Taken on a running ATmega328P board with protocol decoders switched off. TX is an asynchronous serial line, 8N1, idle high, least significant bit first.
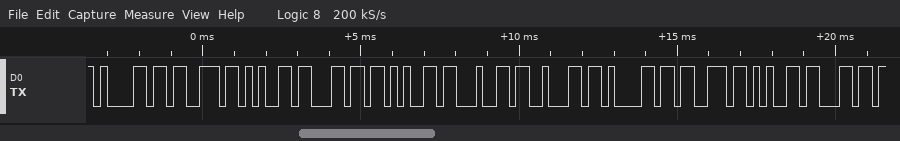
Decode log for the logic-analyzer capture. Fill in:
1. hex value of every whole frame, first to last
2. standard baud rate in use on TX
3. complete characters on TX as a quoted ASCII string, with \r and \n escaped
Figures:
0x61 0x73 0x65 0x6C 0x65 0x64 0x62 0x61 0x73 0x65 0x6C
4800 baud
"aseledbasel"
